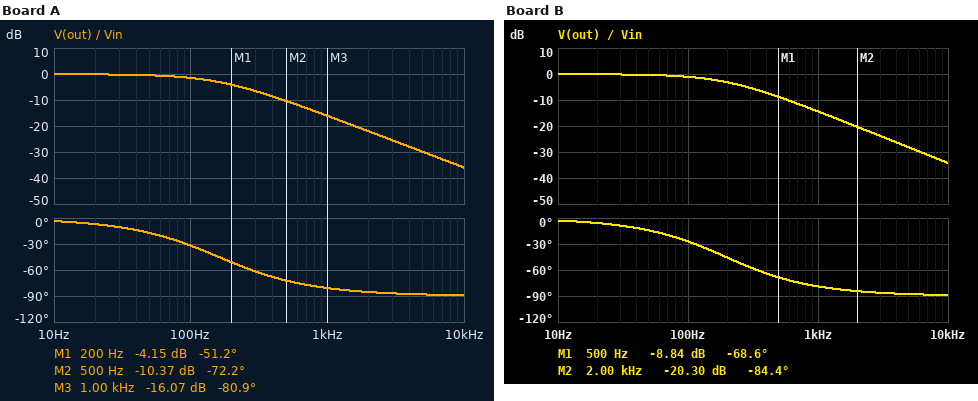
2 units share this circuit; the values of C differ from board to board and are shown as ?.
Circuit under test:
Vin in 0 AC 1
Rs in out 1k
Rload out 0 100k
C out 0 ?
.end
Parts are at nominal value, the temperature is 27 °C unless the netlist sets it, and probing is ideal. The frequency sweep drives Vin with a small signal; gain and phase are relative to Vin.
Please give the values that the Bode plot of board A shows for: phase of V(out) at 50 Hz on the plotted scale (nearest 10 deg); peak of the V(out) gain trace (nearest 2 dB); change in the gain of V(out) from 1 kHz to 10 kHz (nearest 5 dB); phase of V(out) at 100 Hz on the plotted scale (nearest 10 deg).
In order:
-20 deg
0 dB
-20 dB
-30 deg
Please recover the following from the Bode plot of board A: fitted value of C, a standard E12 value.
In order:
1 µF
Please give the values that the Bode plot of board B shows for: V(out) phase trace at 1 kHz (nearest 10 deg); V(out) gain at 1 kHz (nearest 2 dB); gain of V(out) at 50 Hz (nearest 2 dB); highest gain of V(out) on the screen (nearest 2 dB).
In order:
-80 deg
-14 dB
0 dB
0 dB
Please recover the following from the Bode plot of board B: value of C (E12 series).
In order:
820 nF
